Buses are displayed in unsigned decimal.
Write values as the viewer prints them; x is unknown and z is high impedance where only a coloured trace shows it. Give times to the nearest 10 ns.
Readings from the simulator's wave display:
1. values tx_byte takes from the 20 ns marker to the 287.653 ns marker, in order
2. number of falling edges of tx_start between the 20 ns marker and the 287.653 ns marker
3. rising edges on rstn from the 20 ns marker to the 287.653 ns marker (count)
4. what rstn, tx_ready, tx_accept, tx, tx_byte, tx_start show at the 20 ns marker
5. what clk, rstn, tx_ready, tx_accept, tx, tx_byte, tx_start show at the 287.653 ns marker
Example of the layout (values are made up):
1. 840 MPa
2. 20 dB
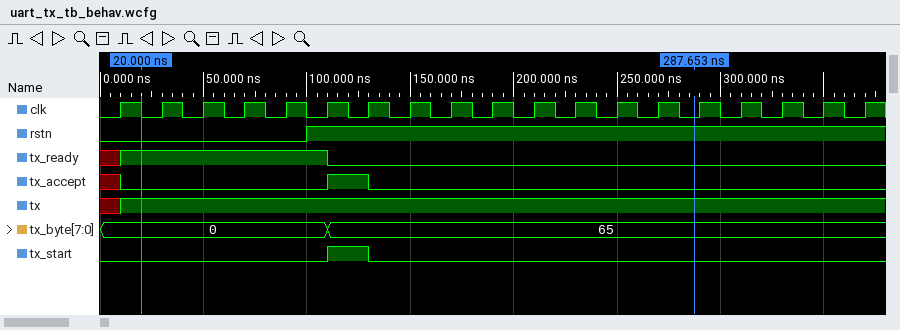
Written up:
1. 0, 65
2. 1
3. 1
4. rstn=0, tx_ready=1, tx_accept=0, tx=1, tx_byte=0, tx_start=0
5. clk=0, rstn=1, tx_ready=0, tx_accept=0, tx=1, tx_byte=65, tx_start=0
